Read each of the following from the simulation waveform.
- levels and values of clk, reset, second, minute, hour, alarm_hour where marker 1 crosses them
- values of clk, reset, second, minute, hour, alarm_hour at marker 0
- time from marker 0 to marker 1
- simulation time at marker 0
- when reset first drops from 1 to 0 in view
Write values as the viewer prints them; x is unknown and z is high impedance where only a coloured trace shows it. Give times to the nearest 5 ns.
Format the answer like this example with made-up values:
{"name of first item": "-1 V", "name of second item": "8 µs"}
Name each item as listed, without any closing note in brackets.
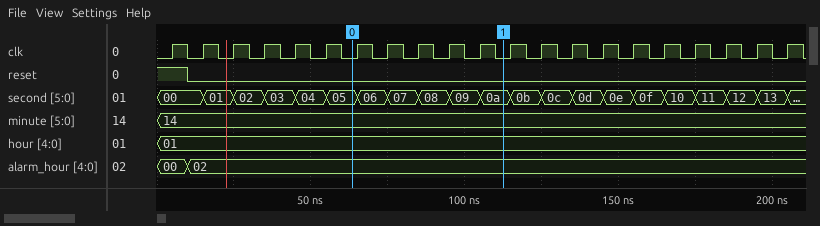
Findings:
{"levels and values of clk, reset, second, minute, hour, alarm_hour where marker 1 crosses them": "clk=0, reset=0, second=0a, minute=14, hour=01, alarm_hour=02", "values of clk, reset, second, minute, hour, alarm_hour at marker 0": "clk=0, reset=0, second=05, minute=14, hour=01, alarm_hour=02", "time from marker 0 to marker 1": "50 ns", "simulation time at marker 0": "65 ns", "when reset first drops from 1 to 0 in view": "10 ns"}
